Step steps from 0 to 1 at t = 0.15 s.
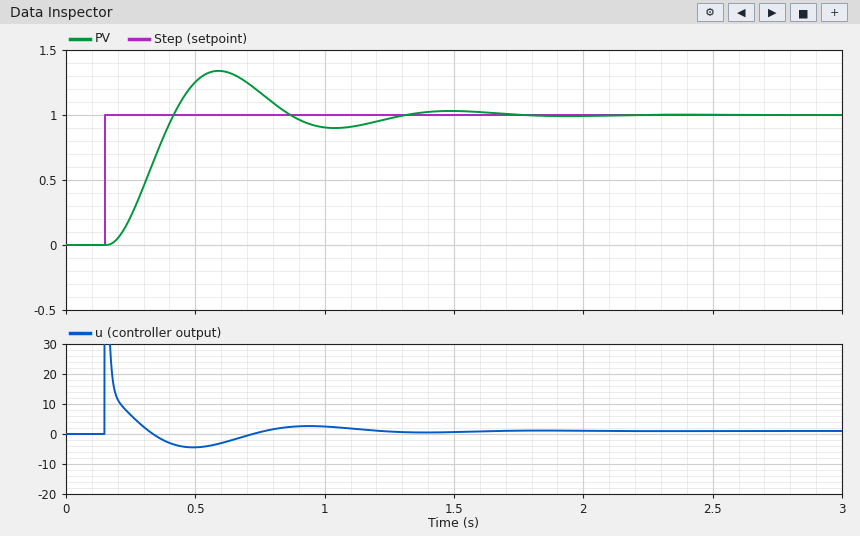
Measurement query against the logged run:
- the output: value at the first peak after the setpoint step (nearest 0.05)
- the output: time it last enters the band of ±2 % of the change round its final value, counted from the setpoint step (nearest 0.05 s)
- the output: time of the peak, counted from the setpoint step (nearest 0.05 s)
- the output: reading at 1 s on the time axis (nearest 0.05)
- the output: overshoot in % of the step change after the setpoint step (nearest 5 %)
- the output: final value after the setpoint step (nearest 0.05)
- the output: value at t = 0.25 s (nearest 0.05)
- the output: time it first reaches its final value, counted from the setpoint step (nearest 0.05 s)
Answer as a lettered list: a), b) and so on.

a) 1.35
b) 1.45 s
c) 0.45 s
d) 0.90
e) 35 %
f) 1.00
g) 0.20
h) 0.25 s
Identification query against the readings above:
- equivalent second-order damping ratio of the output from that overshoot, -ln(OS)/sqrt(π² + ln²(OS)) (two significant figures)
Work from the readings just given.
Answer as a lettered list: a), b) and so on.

a) 0.32
